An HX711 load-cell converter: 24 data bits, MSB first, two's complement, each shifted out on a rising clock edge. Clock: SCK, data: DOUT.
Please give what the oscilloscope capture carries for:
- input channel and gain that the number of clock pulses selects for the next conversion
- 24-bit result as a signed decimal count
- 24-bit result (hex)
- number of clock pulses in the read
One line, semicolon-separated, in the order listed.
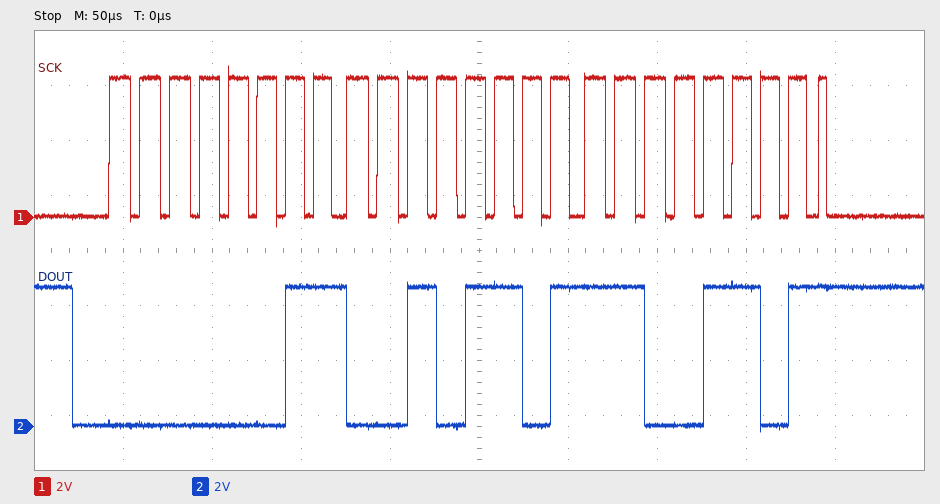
channel A, gain 128; 208333; 0x032DCD; 25
